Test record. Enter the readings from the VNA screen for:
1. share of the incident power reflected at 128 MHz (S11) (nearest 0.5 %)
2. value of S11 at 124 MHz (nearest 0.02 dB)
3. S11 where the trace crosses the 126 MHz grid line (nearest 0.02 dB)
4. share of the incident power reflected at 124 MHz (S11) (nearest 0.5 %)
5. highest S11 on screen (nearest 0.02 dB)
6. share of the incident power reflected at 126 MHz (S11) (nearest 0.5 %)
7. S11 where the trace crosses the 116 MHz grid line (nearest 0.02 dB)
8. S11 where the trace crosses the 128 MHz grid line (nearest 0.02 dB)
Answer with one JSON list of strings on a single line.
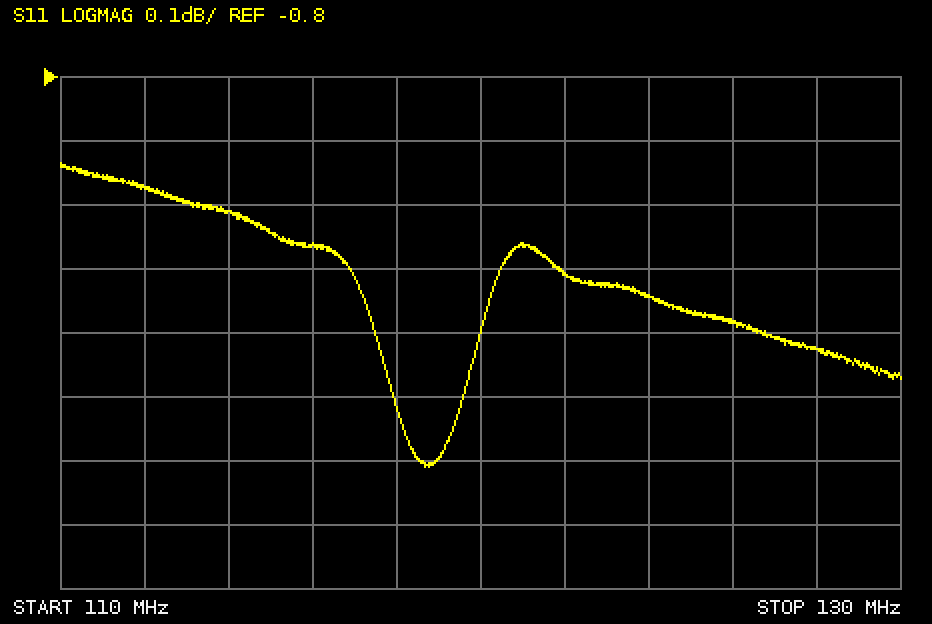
["75.5 %", "-1.14 dB", "-1.18 dB", "77.0 %", "-0.94 dB", "76.0 %", "-1.06 dB", "-1.22 dB"]
